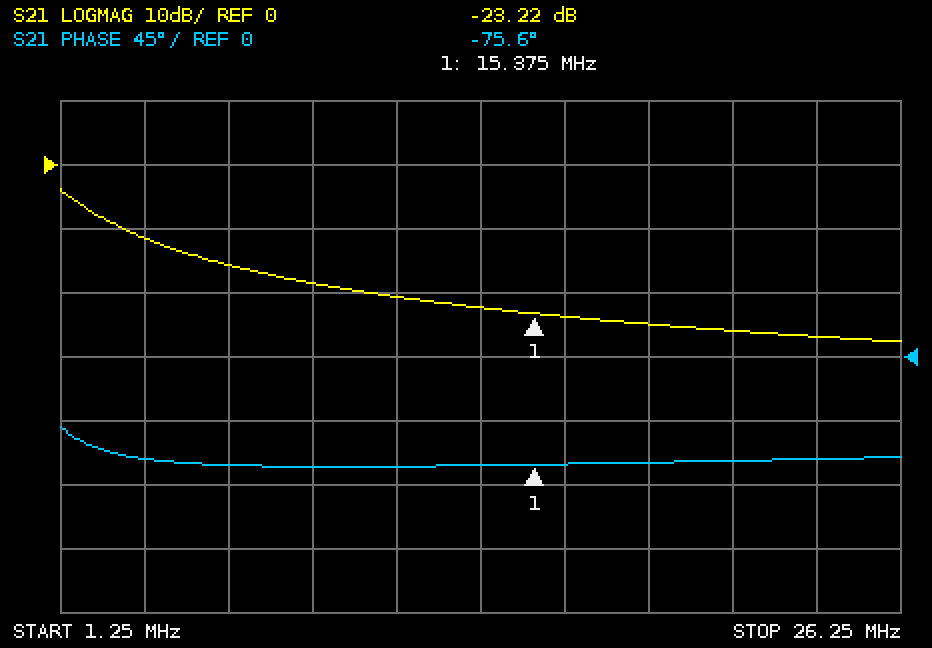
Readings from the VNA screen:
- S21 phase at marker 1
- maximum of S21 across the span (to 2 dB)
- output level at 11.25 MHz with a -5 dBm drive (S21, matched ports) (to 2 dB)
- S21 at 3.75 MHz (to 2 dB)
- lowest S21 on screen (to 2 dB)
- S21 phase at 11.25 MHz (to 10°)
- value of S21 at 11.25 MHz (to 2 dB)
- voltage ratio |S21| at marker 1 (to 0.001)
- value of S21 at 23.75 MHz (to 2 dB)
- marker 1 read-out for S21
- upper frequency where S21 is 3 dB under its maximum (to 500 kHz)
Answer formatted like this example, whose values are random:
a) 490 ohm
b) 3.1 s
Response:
a) -75.6°
b) -4 dB
c) -26 dBm
d) -12 dB
e) -28 dB
f) -80°
g) -20 dB
h) 0.069
i) -26 dB
j) -23.22 dB
k) 2.0 MHz
